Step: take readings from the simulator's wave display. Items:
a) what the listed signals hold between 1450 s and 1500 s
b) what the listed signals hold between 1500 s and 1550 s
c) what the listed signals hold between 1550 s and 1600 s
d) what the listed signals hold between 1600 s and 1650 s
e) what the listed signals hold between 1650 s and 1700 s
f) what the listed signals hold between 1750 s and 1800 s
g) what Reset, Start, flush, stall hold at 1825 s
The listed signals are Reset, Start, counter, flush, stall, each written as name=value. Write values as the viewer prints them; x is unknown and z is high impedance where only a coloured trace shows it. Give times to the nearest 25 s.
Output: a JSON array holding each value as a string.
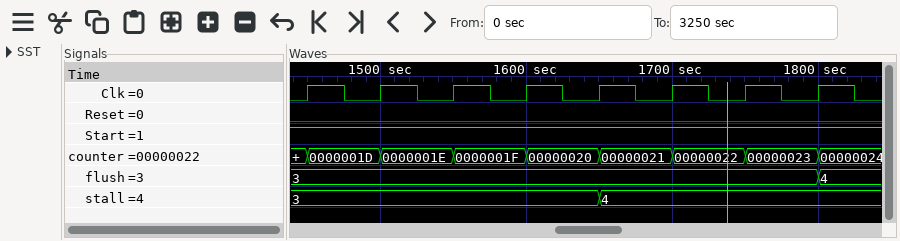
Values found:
["Reset=0, Start=1, counter=0000001D, flush=3, stall=3", "Reset=0, Start=1, counter=0000001E, flush=3, stall=3", "Reset=0, Start=1, counter=0000001F, flush=3, stall=3", "Reset=0, Start=1, counter=00000020, flush=3, stall=3", "Reset=0, Start=1, counter=00000021, flush=3, stall=4", "Reset=0, Start=1, counter=00000023, flush=3, stall=4", "Reset=0, Start=1, flush=4, stall=4"]
